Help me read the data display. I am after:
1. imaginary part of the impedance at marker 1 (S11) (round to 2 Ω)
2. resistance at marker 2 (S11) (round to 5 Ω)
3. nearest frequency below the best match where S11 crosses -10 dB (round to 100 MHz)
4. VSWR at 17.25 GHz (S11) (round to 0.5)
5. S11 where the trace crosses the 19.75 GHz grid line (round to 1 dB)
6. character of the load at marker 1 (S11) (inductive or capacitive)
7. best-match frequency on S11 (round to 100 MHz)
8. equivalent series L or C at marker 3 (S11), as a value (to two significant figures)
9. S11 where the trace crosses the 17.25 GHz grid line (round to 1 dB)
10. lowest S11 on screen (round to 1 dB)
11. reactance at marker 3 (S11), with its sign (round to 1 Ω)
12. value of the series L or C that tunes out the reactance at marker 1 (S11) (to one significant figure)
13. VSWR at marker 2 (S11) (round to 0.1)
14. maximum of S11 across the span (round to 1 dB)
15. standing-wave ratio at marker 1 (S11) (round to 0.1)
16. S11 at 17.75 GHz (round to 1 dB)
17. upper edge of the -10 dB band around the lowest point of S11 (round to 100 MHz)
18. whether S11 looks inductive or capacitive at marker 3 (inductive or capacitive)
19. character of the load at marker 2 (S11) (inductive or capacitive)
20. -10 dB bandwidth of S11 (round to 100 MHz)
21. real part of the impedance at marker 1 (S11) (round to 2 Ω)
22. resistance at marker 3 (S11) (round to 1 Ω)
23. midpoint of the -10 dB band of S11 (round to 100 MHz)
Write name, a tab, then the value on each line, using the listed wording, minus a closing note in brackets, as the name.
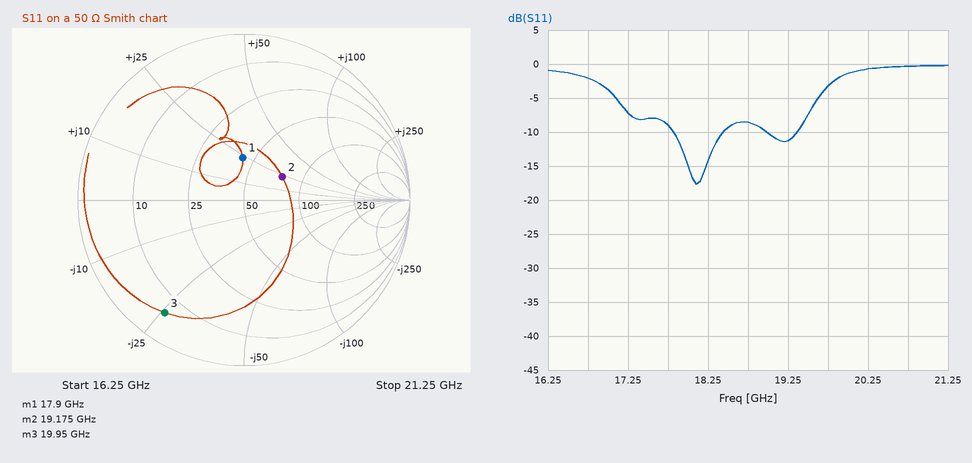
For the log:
imaginary part of the impedance at marker 1 (S11)	+24 Ω
resistance at marker 2 (S11)	75 Ω
nearest frequency below the best match where S11 crosses -10 dB	17.8 GHz
VSWR at 17.25 GHz (S11)	2.5
S11 where the trace crosses the 19.75 GHz grid line	-3 dB
character of the load at marker 1 (S11)	inductive
best-match frequency on S11	18.1 GHz
equivalent series L or C at marker 3 (S11), as a value	310 fF
S11 where the trace crosses the 17.25 GHz grid line	-7 dB
lowest S11 on screen	-18 dB
reactance at marker 3 (S11), with its sign	-26 Ω
value of the series L or C that tunes out the reactance at marker 1 (S11)	400 fF
VSWR at marker 2 (S11)	1.7
maximum of S11 across the span	0 dB
standing-wave ratio at marker 1 (S11)	1.7
S11 at 17.75 GHz	-9 dB
upper edge of the -10 dB band around the lowest point of S11	18.4 GHz
whether S11 looks inductive or capacitive at marker 3	capacitive
character of the load at marker 2 (S11)	inductive
-10 dB bandwidth of S11	600 MHz
real part of the impedance at marker 1 (S11)	44 Ω
resistance at marker 3 (S11)	6 Ω
midpoint of the -10 dB band of S11	18.1 GHz
